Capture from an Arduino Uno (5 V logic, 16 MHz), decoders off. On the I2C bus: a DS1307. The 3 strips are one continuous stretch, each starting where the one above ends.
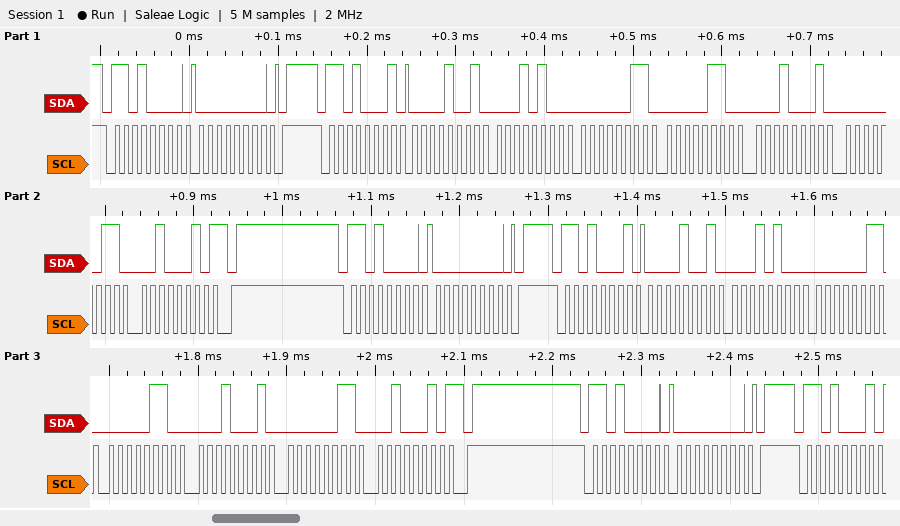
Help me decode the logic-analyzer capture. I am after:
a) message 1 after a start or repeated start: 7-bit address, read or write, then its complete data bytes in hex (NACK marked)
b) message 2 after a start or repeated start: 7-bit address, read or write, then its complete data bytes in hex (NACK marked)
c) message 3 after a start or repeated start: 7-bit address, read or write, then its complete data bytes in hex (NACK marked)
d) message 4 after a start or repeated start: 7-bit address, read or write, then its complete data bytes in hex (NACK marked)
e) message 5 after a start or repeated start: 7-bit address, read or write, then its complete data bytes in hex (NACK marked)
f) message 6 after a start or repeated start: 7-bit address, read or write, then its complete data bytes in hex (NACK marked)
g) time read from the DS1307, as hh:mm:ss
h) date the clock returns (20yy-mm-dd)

0x68 write: 00
0x68 read: 09 14 03 06 11 03 22 NACK
0x68 write: 00
0x68 read: 09 14 03 06 11 03 22 NACK
0x68 write: 00
0x68 read
03:14:09
2022-03-11
